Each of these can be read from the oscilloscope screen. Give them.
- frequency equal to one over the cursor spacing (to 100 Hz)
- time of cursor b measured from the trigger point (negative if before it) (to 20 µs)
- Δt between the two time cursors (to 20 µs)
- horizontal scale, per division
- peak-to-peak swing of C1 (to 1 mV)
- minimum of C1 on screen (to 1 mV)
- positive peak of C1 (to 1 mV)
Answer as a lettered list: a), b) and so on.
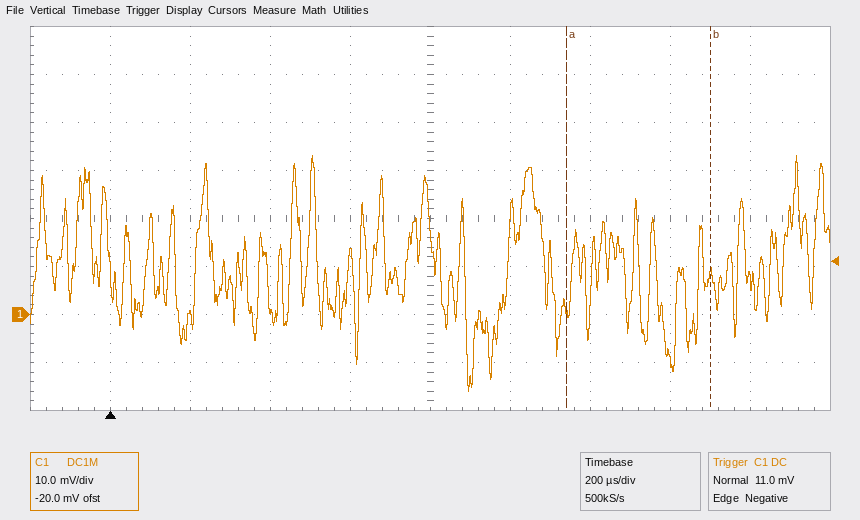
a) 2.8 kHz
b) +1.50 ms
c) 360 µs
d) 200 µs
e) 49 mV
f) -16 mV
g) 33 mV
